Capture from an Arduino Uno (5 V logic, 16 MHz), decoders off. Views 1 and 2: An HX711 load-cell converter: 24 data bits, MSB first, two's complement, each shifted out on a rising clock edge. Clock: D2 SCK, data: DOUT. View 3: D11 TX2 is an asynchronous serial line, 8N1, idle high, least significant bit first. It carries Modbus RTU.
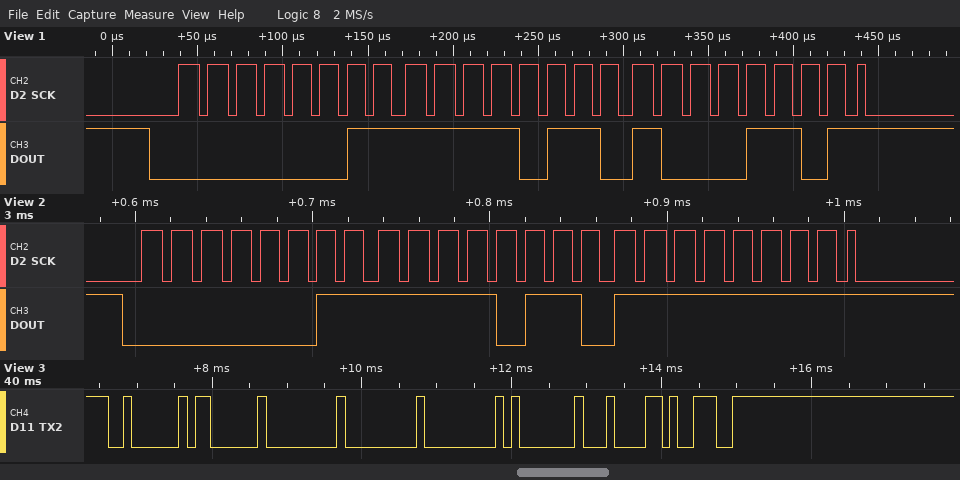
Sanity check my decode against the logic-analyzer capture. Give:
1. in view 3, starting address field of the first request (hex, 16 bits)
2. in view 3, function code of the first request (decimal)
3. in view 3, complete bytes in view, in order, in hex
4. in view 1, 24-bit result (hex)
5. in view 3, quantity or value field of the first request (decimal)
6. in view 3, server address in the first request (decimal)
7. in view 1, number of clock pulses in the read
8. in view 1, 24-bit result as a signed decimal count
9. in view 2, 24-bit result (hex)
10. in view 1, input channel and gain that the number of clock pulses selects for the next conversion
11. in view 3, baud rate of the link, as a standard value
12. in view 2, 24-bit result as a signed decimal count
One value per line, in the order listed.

0x0000
3
02 03 00 00 00 01 84 39
0x03F68D
1
2
25
259725
0x03F6FF
channel A, gain 128
9600 baud
259839
